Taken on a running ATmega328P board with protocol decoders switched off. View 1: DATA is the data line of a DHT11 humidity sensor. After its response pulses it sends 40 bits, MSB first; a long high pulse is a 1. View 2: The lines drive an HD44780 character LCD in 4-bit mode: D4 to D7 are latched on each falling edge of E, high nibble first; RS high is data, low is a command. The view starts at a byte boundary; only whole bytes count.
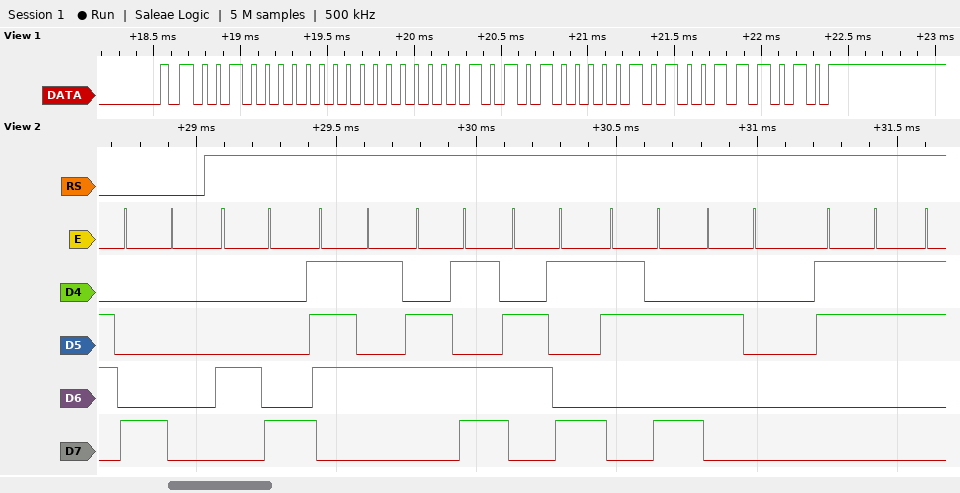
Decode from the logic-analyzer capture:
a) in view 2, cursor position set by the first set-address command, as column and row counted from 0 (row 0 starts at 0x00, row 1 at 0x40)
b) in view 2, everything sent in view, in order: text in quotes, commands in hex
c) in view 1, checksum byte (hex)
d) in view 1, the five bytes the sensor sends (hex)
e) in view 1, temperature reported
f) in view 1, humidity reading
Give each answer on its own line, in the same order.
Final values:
column 0, row 0
0x80 "Humi: 3"
0x3A
20 00 15 05 3A
21.5 °C
32 %
